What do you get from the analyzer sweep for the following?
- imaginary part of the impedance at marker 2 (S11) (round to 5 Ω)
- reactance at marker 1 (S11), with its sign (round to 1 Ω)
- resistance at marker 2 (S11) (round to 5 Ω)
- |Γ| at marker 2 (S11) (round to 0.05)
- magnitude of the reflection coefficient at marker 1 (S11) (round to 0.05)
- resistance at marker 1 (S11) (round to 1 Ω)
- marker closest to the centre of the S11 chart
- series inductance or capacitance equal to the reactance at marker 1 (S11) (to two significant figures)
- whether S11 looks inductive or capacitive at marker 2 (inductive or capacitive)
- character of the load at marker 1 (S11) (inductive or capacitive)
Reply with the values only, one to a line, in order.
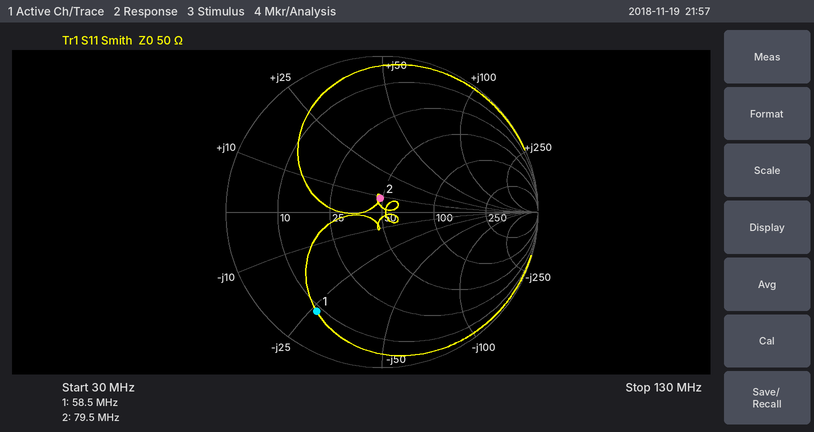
+10 Ω
-26 Ω
50 Ω
0.10
0.75
9 Ω
marker 2
100 pF
inductive
capacitive
